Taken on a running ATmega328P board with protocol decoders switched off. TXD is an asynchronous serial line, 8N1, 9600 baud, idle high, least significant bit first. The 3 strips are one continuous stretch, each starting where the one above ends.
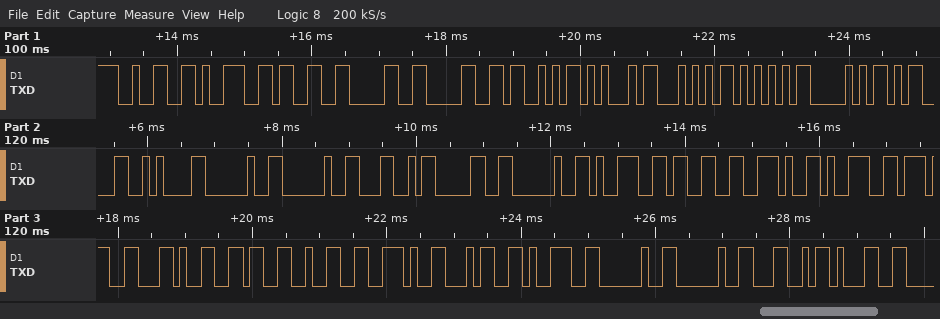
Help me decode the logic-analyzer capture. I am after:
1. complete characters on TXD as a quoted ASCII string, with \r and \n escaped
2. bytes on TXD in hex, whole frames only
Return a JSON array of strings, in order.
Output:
["\"29300SETUP\\r\\n  L0 93.97,62.49  L1\"", "32 39 33 30 30 53 45 54 55 50 0D 0A 20 20 4C 30 20 39 33 2E 39 37 2C 36 32 2E 34 39 20 20 4C 31"]
